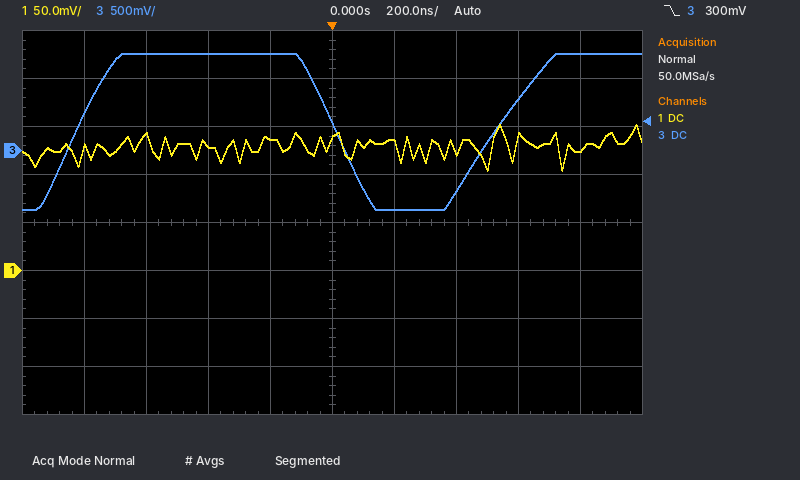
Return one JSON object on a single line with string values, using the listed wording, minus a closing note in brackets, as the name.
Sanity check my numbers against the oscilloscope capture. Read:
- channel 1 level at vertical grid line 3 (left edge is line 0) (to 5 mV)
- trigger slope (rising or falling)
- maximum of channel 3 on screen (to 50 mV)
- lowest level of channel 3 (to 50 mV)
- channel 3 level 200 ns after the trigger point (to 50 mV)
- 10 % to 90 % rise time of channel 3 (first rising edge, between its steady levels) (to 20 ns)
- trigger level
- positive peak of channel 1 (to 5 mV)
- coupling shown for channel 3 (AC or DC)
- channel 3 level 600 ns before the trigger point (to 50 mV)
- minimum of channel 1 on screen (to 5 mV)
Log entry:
{"channel 1 level at vertical grid line 3 (left edge is line 0)": "130 mV", "trigger slope": "falling", "maximum of channel 3 on screen": "1.00 V", "lowest level of channel 3": "-600 mV", "channel 3 level 200 ns after the trigger point": "-600 mV", "10 % to 90 % rise time of channel 3 (first rising edge, between its steady levels)": "200 ns", "trigger level": "300 mV", "positive peak of channel 1": "150 mV", "coupling shown for channel 3": "DC", "channel 3 level 600 ns before the trigger point": "1.00 V", "minimum of channel 1 on screen": "105 mV"}
